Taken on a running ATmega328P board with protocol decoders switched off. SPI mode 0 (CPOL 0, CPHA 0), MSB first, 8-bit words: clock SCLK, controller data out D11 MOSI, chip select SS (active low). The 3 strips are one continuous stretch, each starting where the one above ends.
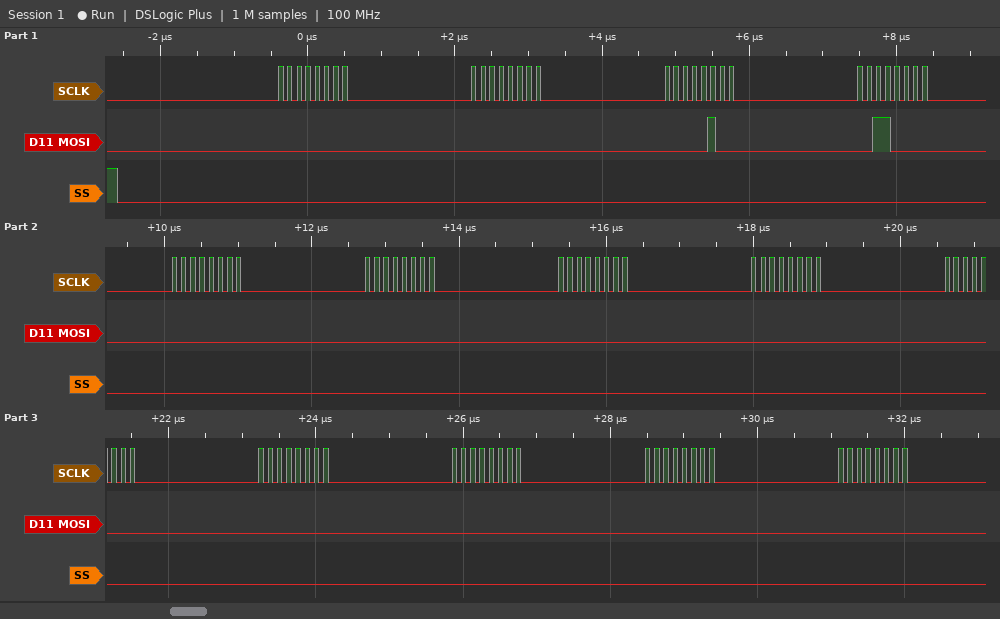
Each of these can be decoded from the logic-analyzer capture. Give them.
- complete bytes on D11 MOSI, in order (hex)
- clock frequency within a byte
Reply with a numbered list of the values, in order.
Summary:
1. 0x00 0x00 0x04 0x30 0x00 0x00 0x00 0x00 0x00 0x00 0x00 0x00 0x00
2. 8 MHz
